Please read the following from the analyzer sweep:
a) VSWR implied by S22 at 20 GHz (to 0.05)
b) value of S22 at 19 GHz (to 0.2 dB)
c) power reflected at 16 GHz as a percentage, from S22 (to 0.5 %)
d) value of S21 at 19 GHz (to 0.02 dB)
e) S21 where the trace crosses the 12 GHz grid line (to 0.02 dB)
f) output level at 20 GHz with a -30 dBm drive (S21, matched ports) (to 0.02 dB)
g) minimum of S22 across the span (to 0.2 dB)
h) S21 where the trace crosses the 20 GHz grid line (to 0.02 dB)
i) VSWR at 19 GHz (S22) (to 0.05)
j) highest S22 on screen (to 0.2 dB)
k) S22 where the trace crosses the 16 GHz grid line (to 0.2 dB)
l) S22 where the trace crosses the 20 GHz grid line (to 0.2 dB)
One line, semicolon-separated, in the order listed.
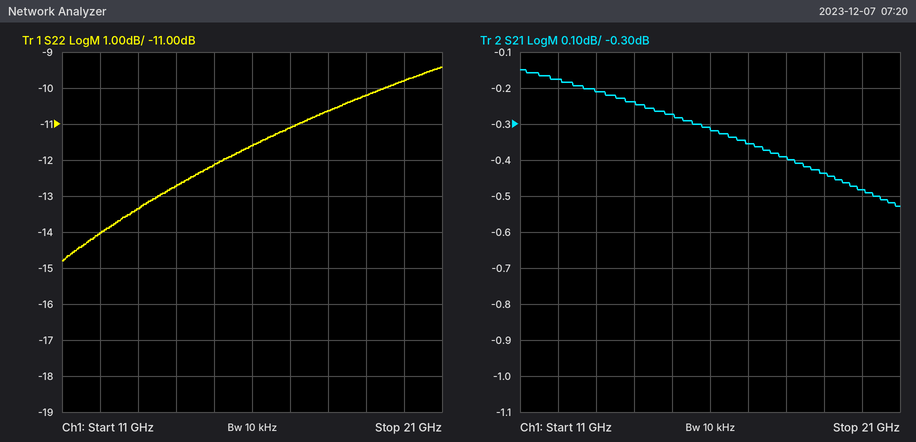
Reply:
1.95; -10.2 dB; 7.0 %; -0.44 dB; -0.18 dB; -30.48 dBm; -14.8 dB; -0.48 dB; 1.90; -9.4 dB; -11.6 dB; -9.8 dB
